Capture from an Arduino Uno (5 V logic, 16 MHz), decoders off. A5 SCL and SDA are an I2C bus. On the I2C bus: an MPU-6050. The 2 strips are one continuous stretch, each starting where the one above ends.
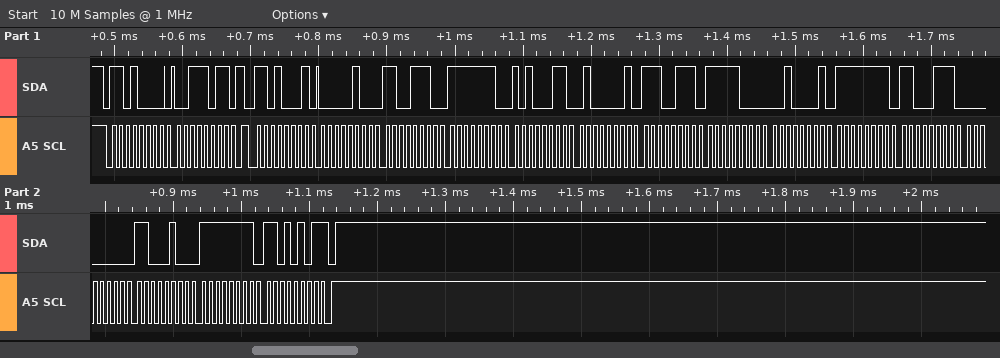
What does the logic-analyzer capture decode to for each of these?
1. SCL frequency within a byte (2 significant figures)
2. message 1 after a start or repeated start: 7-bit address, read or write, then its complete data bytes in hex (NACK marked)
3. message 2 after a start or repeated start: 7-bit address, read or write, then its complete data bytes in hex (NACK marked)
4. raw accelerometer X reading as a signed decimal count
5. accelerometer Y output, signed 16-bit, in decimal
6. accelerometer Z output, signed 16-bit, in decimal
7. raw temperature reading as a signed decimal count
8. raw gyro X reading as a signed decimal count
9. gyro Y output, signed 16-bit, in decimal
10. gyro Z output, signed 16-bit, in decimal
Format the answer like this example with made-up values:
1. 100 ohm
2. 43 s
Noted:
1. 100 kHz
2. 0x68 write: 3B
3. 0x68 read: 04 CE FE A3 41 E7 F8 21 FF C7 00 C4 FF D5 NACK
4. 1230
5. -349
6. 16871
7. -2015
8. -57
9. 196
10. -43
